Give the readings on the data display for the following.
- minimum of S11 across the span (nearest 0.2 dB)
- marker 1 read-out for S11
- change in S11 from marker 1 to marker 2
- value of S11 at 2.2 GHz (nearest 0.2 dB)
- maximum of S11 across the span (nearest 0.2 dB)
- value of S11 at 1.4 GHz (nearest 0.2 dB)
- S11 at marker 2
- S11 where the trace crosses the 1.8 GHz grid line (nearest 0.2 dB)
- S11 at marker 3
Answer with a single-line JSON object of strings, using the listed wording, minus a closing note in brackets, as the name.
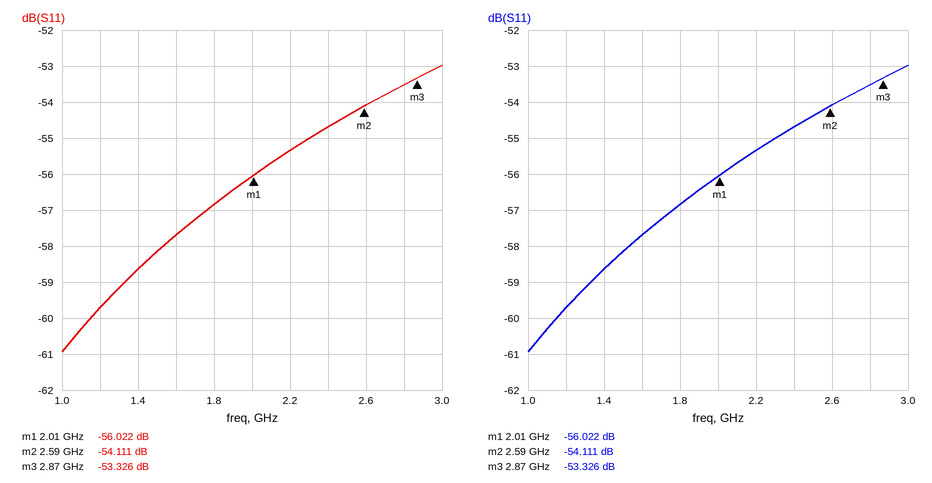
{"minimum of S11 across the span": "-61.0 dB", "marker 1 read-out for S11": "-56.022 dB", "change in S11 from marker 1 to marker 2": "1.911 dB", "value of S11 at 2.2 GHz": "-55.4 dB", "maximum of S11 across the span": "-53.0 dB", "value of S11 at 1.4 GHz": "-58.6 dB", "S11 at marker 2": "-54.111 dB", "S11 where the trace crosses the 1.8 GHz grid line": "-56.8 dB", "S11 at marker 3": "-53.326 dB"}
